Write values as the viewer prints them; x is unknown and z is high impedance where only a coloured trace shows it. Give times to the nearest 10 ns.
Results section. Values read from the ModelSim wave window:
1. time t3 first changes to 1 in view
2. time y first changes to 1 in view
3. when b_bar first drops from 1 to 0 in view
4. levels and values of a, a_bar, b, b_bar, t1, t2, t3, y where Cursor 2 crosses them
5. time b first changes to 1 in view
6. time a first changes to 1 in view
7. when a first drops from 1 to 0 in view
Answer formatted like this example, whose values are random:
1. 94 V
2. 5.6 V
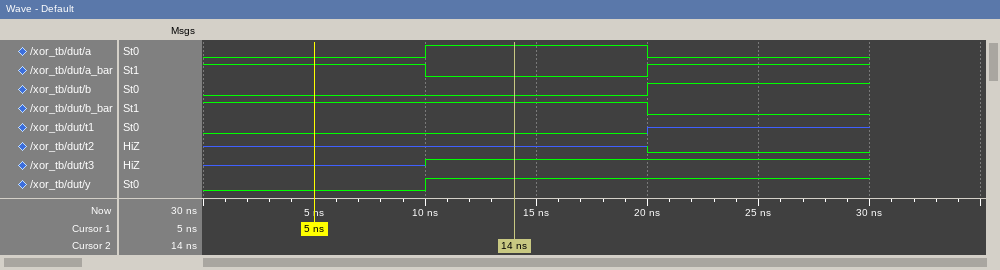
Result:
1. 10 ns
2. 10 ns
3. 20 ns
4. a=1, a_bar=0, b=0, b_bar=1, t1=0, t2=z, t3=1, y=1
5. 20 ns
6. 10 ns
7. 20 ns
